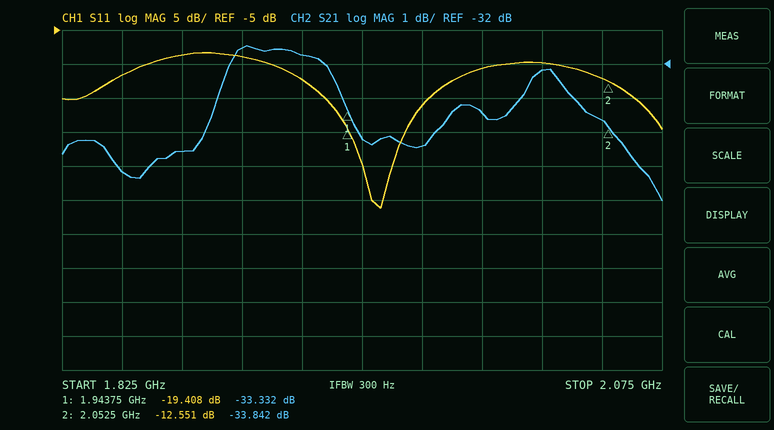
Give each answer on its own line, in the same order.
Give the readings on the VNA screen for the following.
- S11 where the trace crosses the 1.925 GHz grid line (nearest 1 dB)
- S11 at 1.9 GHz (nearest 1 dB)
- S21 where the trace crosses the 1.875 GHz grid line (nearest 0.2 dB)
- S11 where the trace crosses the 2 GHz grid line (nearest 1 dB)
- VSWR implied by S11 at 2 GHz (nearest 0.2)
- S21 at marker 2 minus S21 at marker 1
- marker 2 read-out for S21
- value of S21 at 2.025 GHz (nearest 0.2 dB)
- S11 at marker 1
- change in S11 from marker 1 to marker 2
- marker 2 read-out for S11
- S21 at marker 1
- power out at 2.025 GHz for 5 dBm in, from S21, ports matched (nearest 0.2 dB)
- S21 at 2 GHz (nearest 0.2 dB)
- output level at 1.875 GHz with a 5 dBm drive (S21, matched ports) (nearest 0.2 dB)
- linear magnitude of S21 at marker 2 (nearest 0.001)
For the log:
-12 dB
-9 dB
-34.6 dB
-11 dB
1.8
-0.510 dB
-33.842 dB
-32.2 dB
-19.408 dB
6.857 dB
-12.551 dB
-33.332 dB
-27.2 dBm
-33.4 dB
-29.6 dBm
0.020
